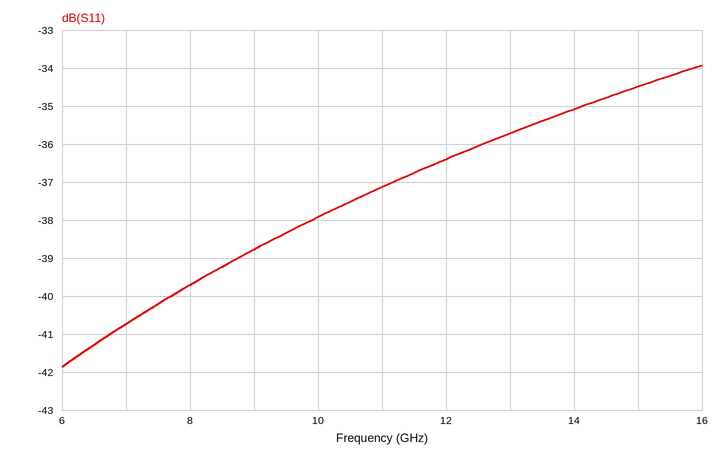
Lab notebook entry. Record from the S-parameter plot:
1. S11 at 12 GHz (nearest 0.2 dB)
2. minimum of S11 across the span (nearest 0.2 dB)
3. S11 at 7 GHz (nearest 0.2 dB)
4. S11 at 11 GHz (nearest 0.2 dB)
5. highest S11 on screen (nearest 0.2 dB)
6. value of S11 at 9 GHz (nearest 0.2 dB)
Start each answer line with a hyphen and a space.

- -36.4 dB
- -41.8 dB
- -40.8 dB
- -37.2 dB
- -34.0 dB
- -38.8 dB
